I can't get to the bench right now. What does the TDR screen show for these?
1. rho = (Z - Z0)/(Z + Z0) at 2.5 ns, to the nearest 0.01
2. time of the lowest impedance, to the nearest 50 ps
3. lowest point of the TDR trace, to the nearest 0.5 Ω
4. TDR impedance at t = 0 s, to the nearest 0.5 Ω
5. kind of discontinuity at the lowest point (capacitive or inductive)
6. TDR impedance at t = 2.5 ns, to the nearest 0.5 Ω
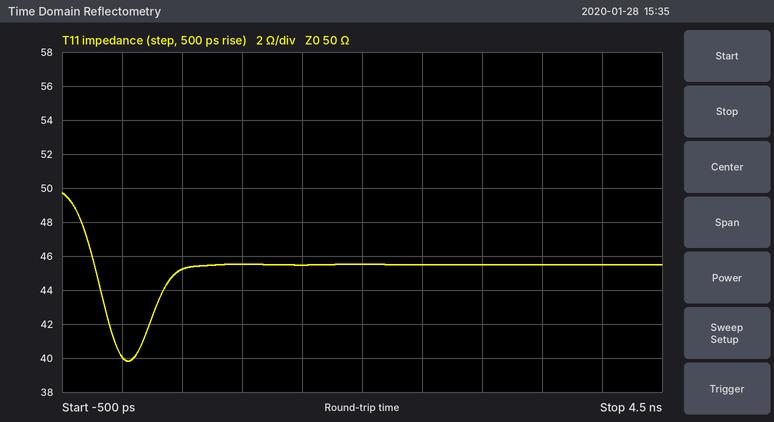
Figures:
-0.05
50 ps
40.0 Ω
40.0 Ω
capacitive
45.5 Ω
